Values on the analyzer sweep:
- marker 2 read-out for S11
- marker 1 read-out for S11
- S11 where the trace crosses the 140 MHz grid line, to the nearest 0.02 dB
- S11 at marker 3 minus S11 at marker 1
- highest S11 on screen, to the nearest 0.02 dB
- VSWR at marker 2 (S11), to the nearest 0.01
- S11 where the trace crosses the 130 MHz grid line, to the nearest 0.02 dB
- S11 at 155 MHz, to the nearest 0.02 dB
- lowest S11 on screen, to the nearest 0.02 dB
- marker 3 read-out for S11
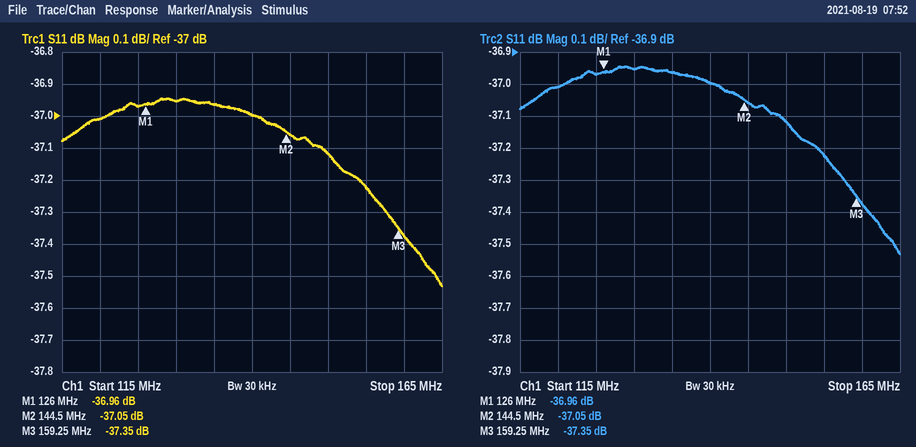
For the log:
-37.05 dB
-36.96 dB
-37.00 dB
-0.39 dB
-36.94 dB
1.03
-36.96 dB
-37.22 dB
-37.54 dB
-37.35 dB
